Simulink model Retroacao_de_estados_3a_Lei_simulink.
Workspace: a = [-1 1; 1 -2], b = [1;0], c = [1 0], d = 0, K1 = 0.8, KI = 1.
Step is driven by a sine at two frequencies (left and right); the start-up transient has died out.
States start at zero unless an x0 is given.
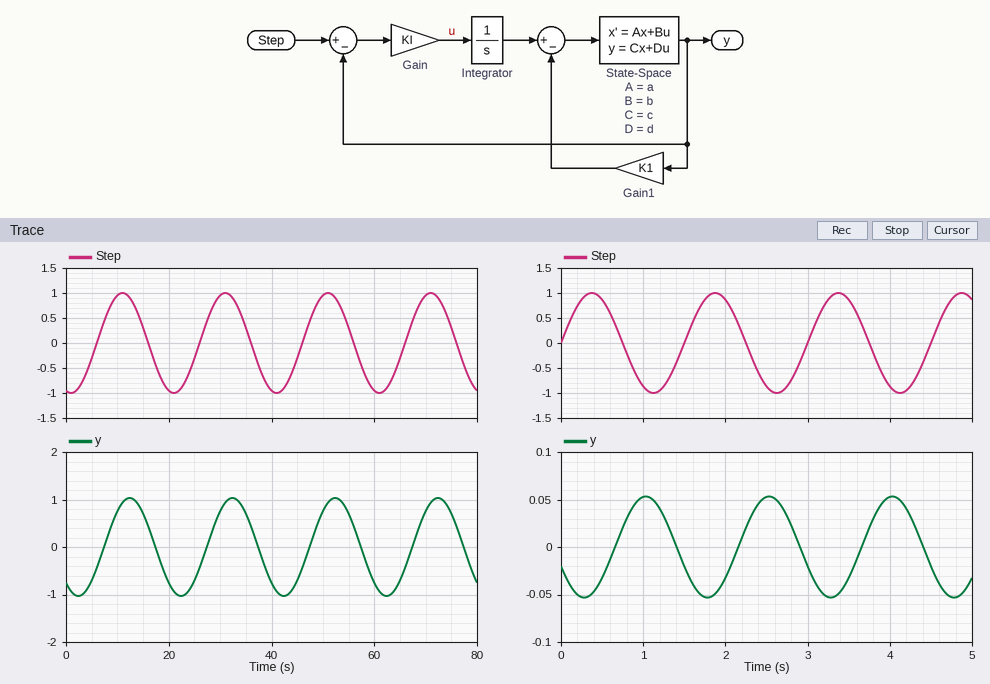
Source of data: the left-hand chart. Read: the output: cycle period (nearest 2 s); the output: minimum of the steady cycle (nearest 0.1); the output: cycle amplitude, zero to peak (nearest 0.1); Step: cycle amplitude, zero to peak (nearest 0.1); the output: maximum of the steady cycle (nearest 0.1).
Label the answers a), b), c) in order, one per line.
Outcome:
a) 20 s
b) -1.0
c) 1.0
d) 1.0
e) 1.0
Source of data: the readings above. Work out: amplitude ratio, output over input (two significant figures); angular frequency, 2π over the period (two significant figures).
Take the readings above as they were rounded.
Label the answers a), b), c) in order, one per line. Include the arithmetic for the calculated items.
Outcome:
a) 1 / 1 = 1.0
b) 2π / 20 = 0.31 rad/s
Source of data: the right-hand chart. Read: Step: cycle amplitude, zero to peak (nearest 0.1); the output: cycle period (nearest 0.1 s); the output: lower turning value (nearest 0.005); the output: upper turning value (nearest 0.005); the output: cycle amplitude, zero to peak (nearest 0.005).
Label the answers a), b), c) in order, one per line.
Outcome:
a) 1.0
b) 1.5 s
c) -0.055
d) 0.055
e) 0.055
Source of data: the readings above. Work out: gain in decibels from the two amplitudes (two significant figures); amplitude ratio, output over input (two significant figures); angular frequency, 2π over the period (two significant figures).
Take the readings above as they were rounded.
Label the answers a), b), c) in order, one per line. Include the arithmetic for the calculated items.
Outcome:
a) 20 log10(0.055 / 1) = -25 dB
b) 0.055 / 1 = 0.055
c) 2π / 1.5 = 4.2 rad/s
